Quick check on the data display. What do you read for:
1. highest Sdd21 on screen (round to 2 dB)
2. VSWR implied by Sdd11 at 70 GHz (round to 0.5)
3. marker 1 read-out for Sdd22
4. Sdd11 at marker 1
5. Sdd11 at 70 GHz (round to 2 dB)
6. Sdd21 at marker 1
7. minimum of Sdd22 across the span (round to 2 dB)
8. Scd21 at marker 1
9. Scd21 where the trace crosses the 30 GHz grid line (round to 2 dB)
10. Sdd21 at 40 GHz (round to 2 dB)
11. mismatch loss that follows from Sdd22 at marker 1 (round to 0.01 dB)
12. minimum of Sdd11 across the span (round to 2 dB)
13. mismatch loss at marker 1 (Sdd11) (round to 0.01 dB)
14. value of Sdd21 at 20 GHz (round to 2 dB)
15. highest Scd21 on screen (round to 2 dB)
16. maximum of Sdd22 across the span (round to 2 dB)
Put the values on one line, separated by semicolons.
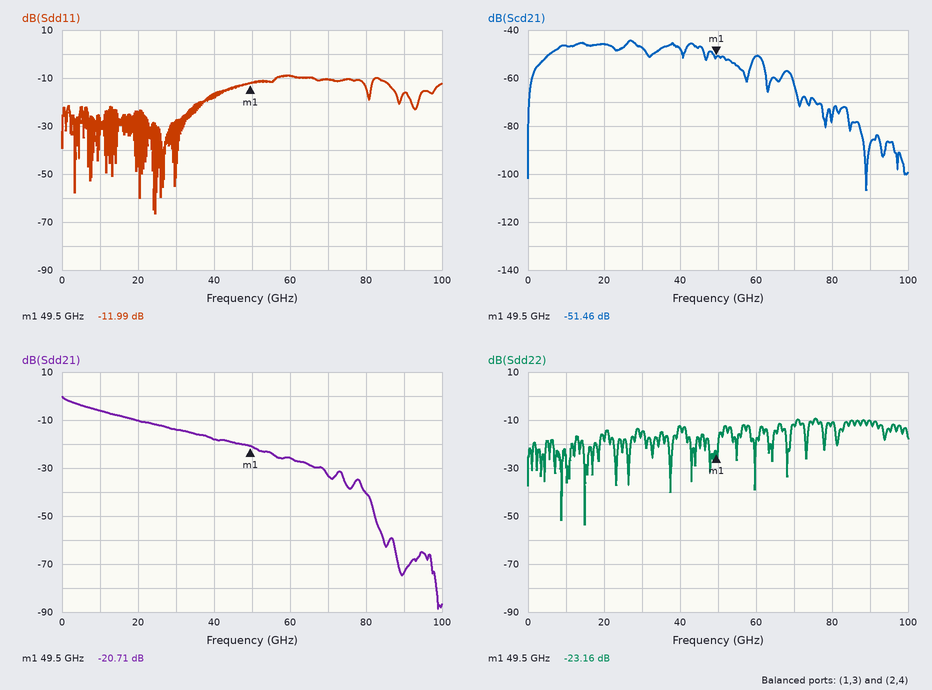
0 dB; 2.0; -23.16 dB; -11.99 dB; -10 dB; -20.71 dB; -54 dB; -51.46 dB; -48 dB; -18 dB; 0.02 dB; -66 dB; 0.28 dB; -10 dB; -44 dB; -10 dB
